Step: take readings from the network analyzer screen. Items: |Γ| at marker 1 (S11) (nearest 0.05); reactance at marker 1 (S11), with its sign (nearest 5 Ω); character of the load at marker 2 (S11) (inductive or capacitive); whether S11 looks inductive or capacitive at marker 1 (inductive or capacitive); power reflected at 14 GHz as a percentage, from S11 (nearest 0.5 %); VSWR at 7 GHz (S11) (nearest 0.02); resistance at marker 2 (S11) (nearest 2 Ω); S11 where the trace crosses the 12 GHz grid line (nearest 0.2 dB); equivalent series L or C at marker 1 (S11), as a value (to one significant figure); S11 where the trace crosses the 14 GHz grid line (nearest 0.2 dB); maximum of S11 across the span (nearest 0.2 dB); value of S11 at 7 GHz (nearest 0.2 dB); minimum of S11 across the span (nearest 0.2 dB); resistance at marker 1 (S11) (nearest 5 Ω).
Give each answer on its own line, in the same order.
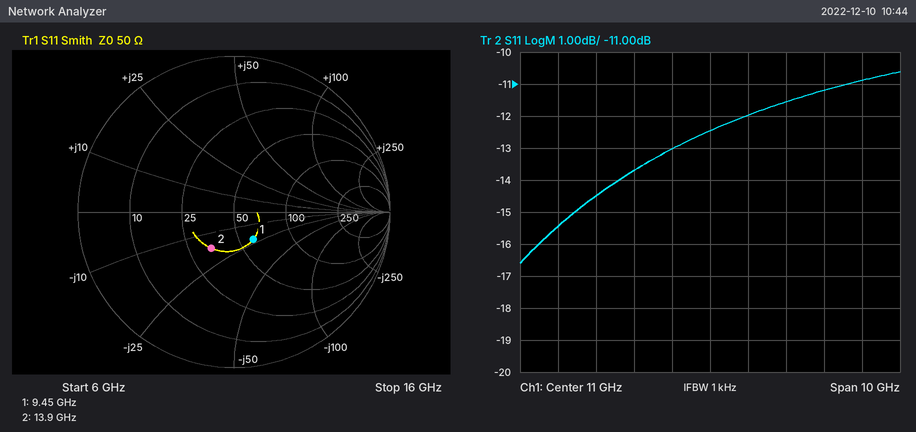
0.20
-20 Ω
capacitive
capacitive
7.5 %
1.40
34 Ω
-12.0 dB
800 fF
-11.2 dB
-10.6 dB
-15.4 dB
-16.6 dB
60 Ω
